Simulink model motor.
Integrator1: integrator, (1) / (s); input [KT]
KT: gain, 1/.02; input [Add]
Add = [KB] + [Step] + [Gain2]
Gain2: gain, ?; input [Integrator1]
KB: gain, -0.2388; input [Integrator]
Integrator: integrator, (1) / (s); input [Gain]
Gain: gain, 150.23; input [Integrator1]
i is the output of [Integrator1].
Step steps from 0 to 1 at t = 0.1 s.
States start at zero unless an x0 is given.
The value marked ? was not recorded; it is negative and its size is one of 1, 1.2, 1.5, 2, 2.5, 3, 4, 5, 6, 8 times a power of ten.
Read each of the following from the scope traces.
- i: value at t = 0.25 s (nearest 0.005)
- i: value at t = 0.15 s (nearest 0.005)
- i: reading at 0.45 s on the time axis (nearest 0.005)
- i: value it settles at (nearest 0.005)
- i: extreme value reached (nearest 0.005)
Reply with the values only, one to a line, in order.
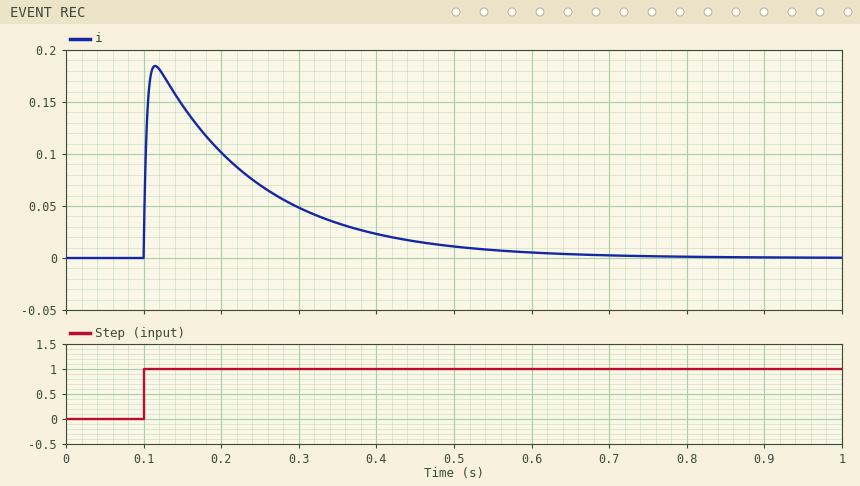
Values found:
0.070
0.145
0.015
0.000
0.185
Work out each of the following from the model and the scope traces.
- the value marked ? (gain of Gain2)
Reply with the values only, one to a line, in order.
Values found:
-5
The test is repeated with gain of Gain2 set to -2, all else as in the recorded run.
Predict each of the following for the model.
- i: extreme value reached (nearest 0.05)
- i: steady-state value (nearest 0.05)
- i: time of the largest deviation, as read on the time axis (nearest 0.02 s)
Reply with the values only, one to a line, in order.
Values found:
0.40
0.00
0.12 s
